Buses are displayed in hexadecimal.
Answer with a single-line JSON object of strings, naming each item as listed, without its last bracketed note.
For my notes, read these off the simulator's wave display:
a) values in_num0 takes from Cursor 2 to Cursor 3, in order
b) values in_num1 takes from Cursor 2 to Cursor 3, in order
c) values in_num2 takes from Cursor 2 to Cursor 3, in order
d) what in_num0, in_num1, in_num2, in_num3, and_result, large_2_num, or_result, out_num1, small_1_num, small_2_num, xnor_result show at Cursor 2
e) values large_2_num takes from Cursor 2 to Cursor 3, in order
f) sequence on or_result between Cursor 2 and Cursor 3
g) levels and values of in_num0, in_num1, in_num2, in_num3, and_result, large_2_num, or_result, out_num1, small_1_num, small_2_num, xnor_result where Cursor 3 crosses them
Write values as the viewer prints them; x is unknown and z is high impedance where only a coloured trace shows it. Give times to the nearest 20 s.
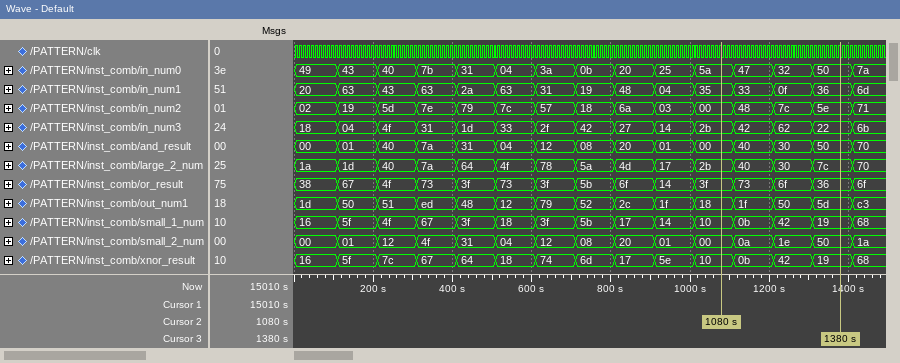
{"values in_num0 takes from Cursor 2 to Cursor 3, in order": "5a, 47, 32, 50", "values in_num1 takes from Cursor 2 to Cursor 3, in order": "35, 33, 0f, 36", "values in_num2 takes from Cursor 2 to Cursor 3, in order": "00, 48, 7c, 5e", "what in_num0, in_num1, in_num2, in_num3, and_result, large_2_num, or_result, out_num1, small_1_num, small_2_num, xnor_result show at Cursor 2": "in_num0=5a, in_num1=35, in_num2=00, in_num3=2b, and_result=00, large_2_num=2b, or_result=3f, out_num1=18, small_1_num=10, small_2_num=00, xnor_result=10", "values large_2_num takes from Cursor 2 to Cursor 3, in order": "2b, 40, 30, 7c", "sequence on or_result between Cursor 2 and Cursor 3": "3f, 73, 6f, 36", "levels and values of in_num0, in_num1, in_num2, in_num3, and_result, large_2_num, or_result, out_num1, small_1_num, small_2_num, xnor_result where Cursor 3 crosses them": "in_num0=50, in_num1=36, in_num2=5e, in_num3=22, and_result=50, large_2_num=7c, or_result=36, out_num1=5d, small_1_num=19, small_2_num=50, xnor_result=19"}
